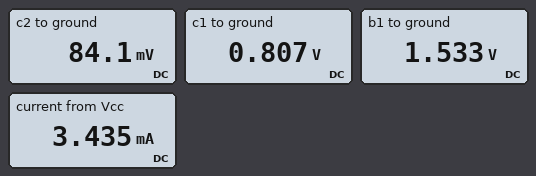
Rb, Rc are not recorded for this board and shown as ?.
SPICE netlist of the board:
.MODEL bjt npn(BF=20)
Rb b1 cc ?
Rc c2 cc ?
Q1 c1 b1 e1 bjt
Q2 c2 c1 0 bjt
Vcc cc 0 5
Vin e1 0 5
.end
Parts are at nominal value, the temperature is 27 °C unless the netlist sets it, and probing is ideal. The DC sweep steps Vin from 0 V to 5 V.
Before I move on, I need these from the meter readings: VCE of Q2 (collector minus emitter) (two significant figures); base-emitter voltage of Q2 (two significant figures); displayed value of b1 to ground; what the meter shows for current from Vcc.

84 mV
810 mV
1.533 V
3.435 mA
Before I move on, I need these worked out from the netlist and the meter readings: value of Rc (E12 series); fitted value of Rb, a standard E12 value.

1.5 kΩ
22 kΩ
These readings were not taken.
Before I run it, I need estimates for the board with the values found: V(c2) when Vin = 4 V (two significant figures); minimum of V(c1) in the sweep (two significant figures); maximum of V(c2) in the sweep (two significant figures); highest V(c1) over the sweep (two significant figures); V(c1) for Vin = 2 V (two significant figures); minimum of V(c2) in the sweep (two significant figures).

84 mV
18 mV
5.0 V
810 mV
810 mV
84 mV
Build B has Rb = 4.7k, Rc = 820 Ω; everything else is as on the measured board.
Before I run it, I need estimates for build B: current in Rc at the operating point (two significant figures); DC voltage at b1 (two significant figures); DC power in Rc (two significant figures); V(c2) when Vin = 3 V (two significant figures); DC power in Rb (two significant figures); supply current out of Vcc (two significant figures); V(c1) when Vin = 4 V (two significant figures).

6.0 mA
1.6 V
30 mW
53 mV
2.5 mW
6.8 mA
830 mV
